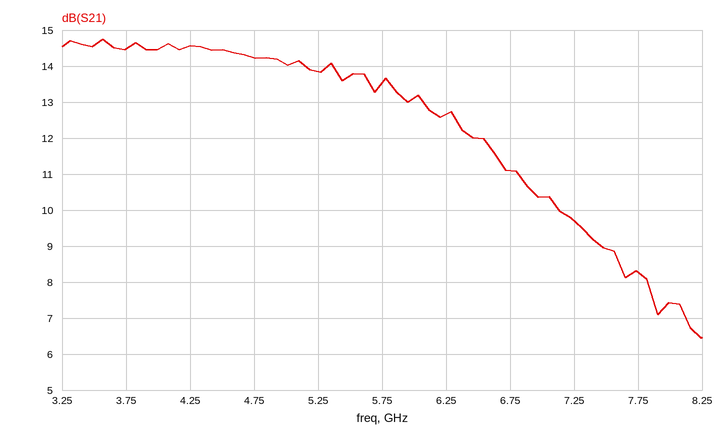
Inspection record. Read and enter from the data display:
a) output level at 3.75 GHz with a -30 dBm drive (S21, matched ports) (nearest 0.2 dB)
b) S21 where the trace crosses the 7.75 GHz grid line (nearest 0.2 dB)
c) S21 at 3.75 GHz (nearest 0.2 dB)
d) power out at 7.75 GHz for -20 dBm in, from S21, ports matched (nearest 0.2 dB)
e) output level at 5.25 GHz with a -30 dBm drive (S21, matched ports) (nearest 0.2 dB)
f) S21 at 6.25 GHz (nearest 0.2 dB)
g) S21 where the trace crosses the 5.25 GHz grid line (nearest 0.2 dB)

-15.6 dBm
8.2 dB
14.4 dB
-11.8 dBm
-16.2 dBm
12.6 dB
13.8 dB
